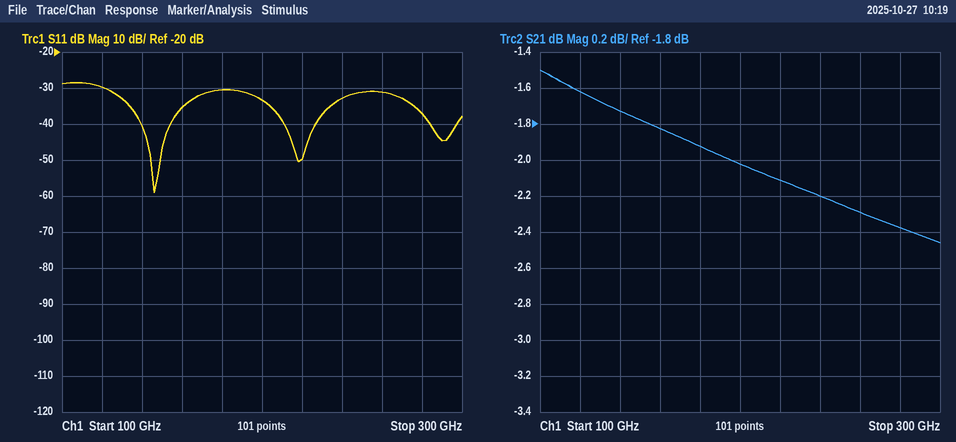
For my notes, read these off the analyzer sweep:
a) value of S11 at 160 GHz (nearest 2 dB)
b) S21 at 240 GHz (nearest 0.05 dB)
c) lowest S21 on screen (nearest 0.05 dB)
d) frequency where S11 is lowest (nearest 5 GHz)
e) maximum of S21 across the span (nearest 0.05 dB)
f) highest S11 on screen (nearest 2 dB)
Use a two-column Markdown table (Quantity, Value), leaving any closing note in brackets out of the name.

| Quantity | Value |
|---|---|
| value of S11 at 160 GHz | -36 dB |
| S21 at 240 GHz | -2.20 dB |
| lowest S21 on screen | -2.45 dB |
| frequency where S11 is lowest | 145 GHz |
| maximum of S21 across the span | -1.50 dB |
| highest S11 on screen | -28 dB |
